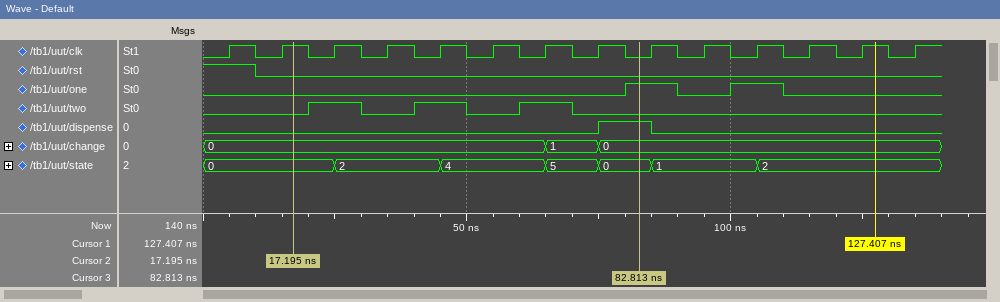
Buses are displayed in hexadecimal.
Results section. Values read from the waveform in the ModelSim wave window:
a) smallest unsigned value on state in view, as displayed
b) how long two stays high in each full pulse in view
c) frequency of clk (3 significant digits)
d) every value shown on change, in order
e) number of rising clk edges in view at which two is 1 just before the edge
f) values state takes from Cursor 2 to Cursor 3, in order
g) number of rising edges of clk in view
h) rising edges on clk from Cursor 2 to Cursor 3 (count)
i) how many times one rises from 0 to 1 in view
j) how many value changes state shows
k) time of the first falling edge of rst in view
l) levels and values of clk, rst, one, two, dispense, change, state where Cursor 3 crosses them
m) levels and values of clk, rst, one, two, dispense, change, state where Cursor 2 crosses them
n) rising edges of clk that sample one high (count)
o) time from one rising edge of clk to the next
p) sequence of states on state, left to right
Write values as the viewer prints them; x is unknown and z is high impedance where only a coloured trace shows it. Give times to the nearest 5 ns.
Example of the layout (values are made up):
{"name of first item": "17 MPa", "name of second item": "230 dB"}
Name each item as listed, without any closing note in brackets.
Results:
{"smallest unsigned value on state in view, as displayed": "0", "how long two stays high in each full pulse in view": "10 ns, 10 ns, 10 ns", "frequency of clk": "100 MHz", "every value shown on change, in order": "0, 1, 0", "number of rising clk edges in view at which two is 1 just before the edge": "3", "values state takes from Cursor 2 to Cursor 3, in order": "0, 2, 4, 5, 0", "number of rising edges of clk in view": "14", "rising edges on clk from Cursor 2 to Cursor 3": "6", "how many times one rises from 0 to 1 in view": "2", "how many value changes state shows": "6", "time of the first falling edge of rst in view": "10 ns", "levels and values of clk, rst, one, two, dispense, change, state where Cursor 3 crosses them": "clk=0, rst=0, one=1, two=0, dispense=1, change=0, state=0", "levels and values of clk, rst, one, two, dispense, change, state where Cursor 2 crosses them": "clk=1, rst=0, one=0, two=0, dispense=0, change=0, state=0", "rising edges of clk that sample one high": "2", "time from one rising edge of clk to the next": "10 ns", "sequence of states on state, left to right": "0, 2, 4, 5, 0, 1, 2"}
